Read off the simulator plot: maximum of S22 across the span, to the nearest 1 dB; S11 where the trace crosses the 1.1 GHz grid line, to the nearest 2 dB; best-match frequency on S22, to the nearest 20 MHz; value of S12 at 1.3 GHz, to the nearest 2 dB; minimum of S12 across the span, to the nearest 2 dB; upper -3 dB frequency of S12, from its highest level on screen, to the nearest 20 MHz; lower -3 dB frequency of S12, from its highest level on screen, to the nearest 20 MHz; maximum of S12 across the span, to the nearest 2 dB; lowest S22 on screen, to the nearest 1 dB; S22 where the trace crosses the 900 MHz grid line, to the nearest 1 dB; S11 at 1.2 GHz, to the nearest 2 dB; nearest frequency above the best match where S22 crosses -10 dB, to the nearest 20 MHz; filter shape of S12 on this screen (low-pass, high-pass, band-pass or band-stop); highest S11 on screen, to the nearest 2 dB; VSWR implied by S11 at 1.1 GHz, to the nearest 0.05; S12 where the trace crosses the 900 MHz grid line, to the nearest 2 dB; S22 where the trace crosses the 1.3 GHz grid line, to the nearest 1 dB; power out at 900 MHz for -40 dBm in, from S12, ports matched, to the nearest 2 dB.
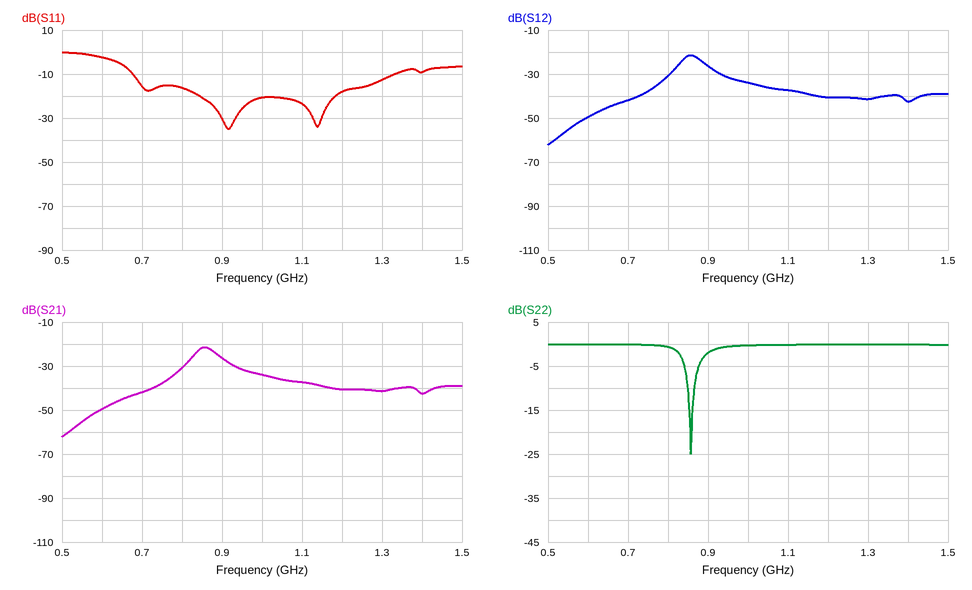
0 dB
-24 dB
860 MHz
-42 dB
-62 dB
880 MHz
840 MHz
-22 dB
-25 dB
-2 dB
-18 dB
860 MHz
band-pass
0 dB
1.15
-26 dB
0 dB
-66 dBm
